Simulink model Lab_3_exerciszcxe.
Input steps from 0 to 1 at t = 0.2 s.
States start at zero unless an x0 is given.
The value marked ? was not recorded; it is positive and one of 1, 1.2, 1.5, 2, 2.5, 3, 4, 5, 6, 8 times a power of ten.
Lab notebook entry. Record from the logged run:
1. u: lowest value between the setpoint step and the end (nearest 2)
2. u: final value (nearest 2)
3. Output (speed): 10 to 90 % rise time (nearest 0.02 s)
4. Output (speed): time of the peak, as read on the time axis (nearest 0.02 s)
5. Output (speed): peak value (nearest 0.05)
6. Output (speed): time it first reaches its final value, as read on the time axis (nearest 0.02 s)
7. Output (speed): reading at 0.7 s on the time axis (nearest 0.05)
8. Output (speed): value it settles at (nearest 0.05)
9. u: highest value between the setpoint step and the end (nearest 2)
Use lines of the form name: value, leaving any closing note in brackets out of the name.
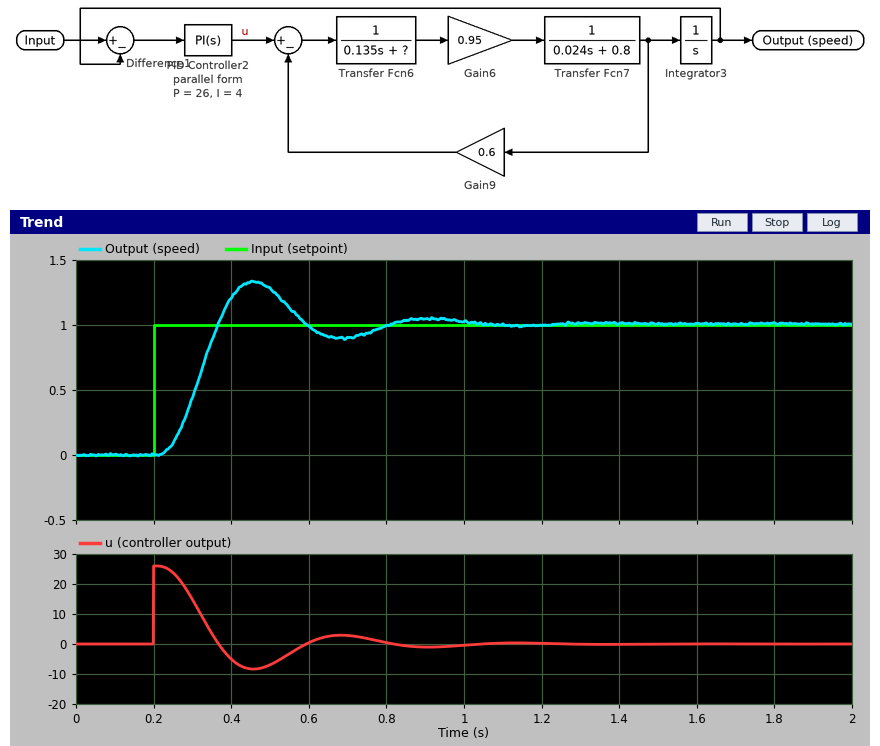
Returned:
u: lowest value between the setpoint step and the end: -8
u: final value: 0
Output (speed): 10 to 90 % rise time: 0.10 s
Output (speed): time of the peak, as read on the time axis: 0.46 s
Output (speed): peak value: 1.35
Output (speed): time it first reaches its final value, as read on the time axis: 0.36 s
Output (speed): reading at 0.7 s on the time axis: 0.90
Output (speed): value it settles at: 1.00
u: highest value between the setpoint step and the end: 26
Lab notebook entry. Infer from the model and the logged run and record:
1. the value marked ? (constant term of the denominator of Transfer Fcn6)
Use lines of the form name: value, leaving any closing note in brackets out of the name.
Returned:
the value marked ?: 1.5
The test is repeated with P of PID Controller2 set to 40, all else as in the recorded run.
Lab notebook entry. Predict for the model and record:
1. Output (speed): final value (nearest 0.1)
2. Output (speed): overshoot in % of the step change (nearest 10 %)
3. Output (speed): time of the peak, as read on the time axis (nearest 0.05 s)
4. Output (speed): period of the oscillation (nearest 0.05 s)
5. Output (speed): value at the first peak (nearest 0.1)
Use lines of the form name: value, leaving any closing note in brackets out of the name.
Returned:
Output (speed): final value: 1.0
Output (speed): overshoot in % of the step change: 50 %
Output (speed): time of the peak, as read on the time axis: 0.40 s
Output (speed): period of the oscillation: 0.35 s
Output (speed): value at the first peak: 1.5
